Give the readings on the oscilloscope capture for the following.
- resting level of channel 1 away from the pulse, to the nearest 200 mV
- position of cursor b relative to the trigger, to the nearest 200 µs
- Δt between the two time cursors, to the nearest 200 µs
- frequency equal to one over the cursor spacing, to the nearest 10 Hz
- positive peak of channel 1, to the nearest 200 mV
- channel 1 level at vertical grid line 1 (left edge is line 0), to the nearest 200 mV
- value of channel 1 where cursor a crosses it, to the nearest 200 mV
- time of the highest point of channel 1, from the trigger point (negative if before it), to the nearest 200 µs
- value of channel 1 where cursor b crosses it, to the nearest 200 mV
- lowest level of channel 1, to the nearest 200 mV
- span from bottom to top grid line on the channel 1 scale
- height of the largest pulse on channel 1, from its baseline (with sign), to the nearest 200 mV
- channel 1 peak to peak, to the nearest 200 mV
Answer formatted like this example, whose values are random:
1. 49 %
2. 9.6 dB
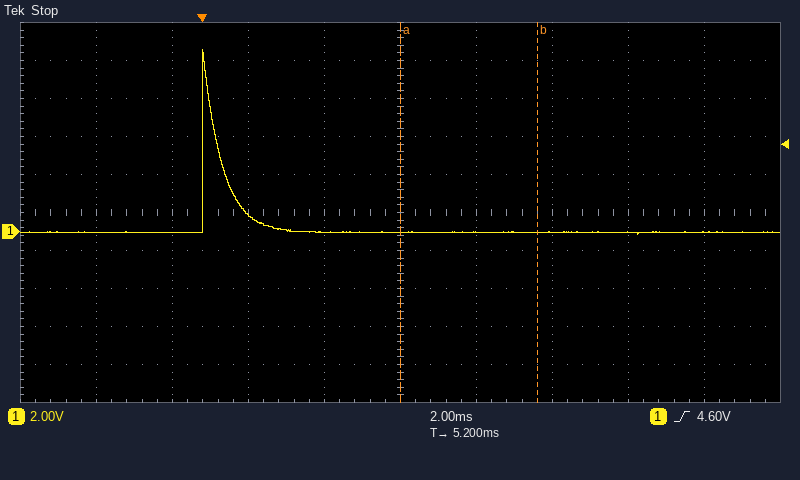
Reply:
1. 0.0 V
2. +8.8 ms
3. 3.6 ms
4. 280 Hz
5. 9.6 V
6. 0.0 V
7. 0.0 V
8. 0.0 ms
9. 0.0 V
10. -200 mV
11. 20 V
12. +9.6 V
13. 9.8 V
